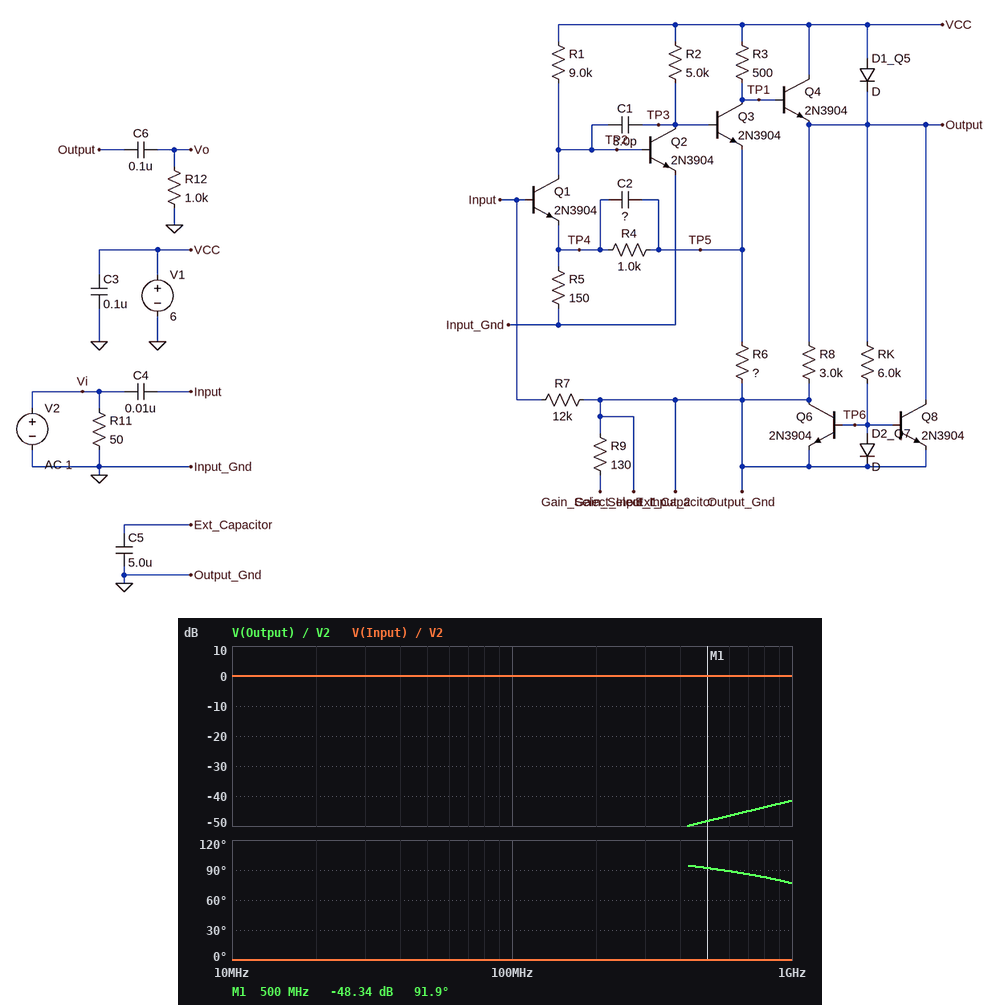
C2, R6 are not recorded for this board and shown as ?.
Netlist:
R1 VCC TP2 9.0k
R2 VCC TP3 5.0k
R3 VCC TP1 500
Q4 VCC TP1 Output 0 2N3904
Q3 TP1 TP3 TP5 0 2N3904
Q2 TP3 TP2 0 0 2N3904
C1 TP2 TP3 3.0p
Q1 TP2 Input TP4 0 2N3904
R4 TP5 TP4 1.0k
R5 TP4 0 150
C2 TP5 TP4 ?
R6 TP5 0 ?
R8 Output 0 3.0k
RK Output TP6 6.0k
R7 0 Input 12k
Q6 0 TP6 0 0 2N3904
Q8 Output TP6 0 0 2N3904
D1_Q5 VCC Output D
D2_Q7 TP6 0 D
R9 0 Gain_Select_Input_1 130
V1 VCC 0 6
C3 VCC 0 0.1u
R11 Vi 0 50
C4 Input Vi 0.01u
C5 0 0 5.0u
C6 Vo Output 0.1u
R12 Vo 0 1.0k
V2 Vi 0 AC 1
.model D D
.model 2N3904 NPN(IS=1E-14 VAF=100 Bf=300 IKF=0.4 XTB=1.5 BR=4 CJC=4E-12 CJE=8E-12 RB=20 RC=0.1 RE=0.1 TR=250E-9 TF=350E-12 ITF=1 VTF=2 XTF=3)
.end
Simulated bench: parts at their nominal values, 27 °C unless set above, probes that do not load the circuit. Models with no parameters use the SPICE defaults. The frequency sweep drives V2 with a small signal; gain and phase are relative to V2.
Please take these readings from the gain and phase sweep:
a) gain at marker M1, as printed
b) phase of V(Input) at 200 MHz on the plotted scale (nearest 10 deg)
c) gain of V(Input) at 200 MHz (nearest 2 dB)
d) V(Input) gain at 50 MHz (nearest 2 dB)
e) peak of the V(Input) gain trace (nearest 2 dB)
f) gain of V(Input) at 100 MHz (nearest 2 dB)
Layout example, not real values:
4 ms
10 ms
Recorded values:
-48.34 dB
0 deg
0 dB
0 dB
0 dB
0 dB
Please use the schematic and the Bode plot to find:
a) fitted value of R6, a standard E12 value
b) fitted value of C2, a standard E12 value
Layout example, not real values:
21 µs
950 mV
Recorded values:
120 Ω
1.2 pF
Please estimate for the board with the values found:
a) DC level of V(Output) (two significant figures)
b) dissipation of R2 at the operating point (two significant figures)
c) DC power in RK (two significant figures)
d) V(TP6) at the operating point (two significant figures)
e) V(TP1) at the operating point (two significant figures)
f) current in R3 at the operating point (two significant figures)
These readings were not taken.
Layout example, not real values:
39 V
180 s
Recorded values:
5.3 V
7.2 mW
3.7 mW
640 mV
6.0 V
5.1 µA
